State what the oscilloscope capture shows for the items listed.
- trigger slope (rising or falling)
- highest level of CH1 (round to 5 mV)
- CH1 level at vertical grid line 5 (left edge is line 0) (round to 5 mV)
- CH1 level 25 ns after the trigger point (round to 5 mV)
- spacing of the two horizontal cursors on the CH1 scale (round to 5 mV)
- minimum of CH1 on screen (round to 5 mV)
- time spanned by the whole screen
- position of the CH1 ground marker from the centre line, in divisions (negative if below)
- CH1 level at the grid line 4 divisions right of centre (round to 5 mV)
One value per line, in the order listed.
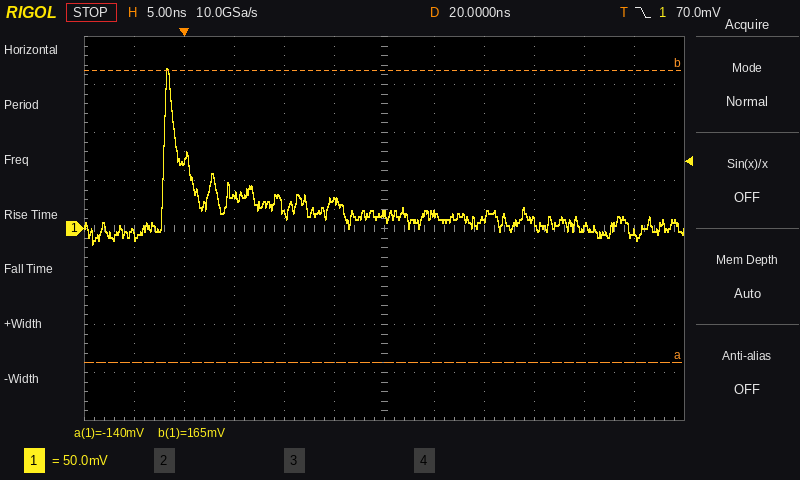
falling
165 mV
30 mV
15 mV
305 mV
-15 mV
60 ns
0.0 div
0 mV
